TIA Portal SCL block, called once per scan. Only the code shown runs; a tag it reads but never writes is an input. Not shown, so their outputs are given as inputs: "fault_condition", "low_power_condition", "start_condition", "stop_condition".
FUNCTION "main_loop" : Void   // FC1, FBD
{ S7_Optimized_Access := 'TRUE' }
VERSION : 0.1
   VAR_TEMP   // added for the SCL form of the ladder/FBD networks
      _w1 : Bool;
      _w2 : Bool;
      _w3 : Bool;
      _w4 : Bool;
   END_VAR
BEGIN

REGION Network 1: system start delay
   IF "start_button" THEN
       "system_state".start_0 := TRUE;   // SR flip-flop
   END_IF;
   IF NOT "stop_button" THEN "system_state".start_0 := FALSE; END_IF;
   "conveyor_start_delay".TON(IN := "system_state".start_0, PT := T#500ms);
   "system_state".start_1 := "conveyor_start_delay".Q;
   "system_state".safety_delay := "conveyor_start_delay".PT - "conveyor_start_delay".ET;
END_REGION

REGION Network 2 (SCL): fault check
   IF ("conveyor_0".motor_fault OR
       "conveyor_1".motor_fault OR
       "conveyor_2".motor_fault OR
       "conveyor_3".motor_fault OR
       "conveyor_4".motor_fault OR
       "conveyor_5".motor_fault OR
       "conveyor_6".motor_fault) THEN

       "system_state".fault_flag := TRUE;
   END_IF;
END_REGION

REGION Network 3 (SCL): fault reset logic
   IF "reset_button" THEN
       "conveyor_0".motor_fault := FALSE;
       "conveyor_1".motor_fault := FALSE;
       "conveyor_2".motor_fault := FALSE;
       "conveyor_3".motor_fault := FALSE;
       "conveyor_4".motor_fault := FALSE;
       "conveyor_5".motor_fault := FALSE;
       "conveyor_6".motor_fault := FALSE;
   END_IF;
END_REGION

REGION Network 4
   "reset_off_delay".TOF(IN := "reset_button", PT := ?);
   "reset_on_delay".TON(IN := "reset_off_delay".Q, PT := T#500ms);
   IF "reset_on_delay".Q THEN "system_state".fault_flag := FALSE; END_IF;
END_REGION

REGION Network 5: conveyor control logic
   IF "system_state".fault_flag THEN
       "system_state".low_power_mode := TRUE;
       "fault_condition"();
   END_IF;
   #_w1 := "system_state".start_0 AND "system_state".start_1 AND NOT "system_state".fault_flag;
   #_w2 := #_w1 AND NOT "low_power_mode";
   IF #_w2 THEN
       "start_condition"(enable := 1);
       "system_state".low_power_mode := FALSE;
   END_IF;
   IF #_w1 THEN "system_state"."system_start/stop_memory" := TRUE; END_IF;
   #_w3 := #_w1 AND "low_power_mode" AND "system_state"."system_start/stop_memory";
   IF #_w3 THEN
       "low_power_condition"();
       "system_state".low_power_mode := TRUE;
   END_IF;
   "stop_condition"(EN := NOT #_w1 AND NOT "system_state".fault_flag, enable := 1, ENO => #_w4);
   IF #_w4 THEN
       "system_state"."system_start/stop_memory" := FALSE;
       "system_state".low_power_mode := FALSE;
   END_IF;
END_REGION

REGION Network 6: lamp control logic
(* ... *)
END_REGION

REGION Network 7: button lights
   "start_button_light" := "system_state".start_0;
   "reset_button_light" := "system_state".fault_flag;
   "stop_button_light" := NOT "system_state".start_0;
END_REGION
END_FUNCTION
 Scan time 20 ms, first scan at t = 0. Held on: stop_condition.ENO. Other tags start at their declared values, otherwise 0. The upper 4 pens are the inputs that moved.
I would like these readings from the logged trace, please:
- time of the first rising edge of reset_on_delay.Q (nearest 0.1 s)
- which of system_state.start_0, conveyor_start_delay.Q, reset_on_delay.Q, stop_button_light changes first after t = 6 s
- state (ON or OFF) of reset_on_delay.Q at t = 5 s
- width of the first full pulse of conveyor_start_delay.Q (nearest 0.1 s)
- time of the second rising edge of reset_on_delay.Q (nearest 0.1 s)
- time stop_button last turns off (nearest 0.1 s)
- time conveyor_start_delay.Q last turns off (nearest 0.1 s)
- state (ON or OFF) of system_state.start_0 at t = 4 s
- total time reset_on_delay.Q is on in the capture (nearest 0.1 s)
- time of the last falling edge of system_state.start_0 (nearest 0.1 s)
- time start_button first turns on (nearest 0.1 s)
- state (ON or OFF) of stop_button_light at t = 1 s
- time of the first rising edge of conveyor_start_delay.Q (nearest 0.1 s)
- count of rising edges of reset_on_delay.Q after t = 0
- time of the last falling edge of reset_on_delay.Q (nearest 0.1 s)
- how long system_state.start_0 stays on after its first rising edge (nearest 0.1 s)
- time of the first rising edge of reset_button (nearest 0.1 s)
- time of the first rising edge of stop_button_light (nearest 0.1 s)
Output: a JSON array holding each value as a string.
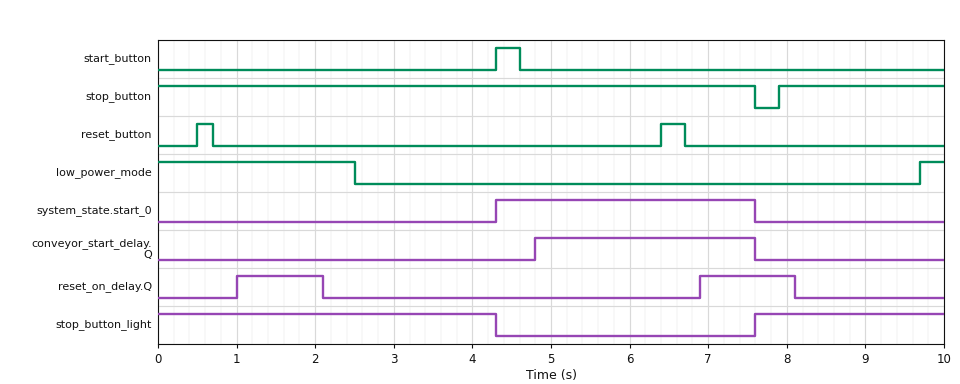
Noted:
["1.0 s", "reset_on_delay.Q", "OFF", "2.8 s", "6.9 s", "7.6 s", "7.6 s", "OFF", "2.3 s", "7.6 s", "4.3 s", "ON", "4.8 s", "2", "8.1 s", "3.3 s", "0.5 s", "7.6 s"]
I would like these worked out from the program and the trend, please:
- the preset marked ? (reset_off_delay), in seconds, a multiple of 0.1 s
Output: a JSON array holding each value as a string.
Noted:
["1.4 s"]
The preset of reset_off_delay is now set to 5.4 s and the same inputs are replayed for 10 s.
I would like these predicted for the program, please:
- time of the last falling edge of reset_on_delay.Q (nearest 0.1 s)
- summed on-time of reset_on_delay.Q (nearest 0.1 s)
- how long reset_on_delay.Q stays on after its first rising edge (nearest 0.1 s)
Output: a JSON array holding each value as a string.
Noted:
["6.1 s", "8.2 s", "5.1 s"]
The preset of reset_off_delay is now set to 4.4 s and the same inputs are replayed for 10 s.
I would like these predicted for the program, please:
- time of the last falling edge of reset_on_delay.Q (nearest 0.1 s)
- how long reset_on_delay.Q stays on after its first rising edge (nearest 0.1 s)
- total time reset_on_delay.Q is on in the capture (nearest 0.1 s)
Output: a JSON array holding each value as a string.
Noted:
["5.1 s", "4.1 s", "7.2 s"]
